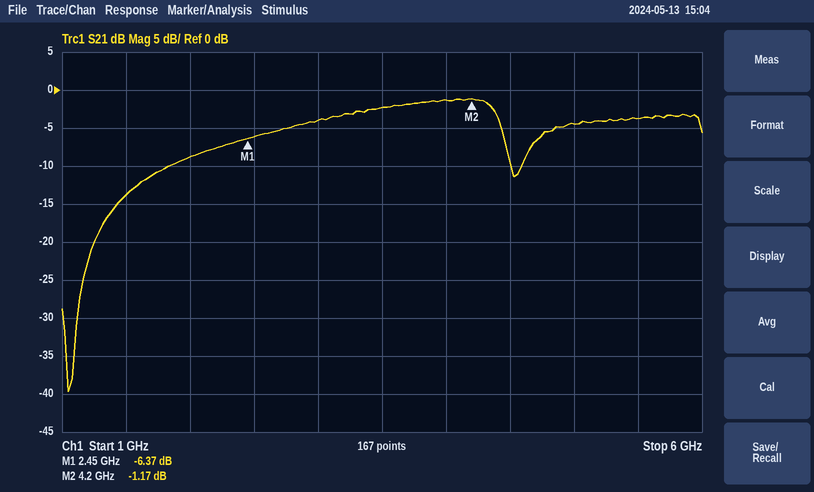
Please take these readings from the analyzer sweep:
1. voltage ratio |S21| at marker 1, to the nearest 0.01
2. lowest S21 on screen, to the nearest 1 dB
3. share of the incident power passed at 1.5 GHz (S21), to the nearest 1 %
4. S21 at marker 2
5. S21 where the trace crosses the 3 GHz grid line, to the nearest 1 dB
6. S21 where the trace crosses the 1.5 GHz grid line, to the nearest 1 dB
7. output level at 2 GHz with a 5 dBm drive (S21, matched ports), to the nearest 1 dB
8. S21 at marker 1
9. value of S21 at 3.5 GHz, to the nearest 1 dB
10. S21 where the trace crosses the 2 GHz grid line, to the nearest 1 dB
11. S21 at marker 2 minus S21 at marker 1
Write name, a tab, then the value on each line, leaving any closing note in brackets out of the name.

voltage ratio |S21| at marker 1, to the nearest 0.01	0.48
lowest S21 on screen, to the nearest 1 dB	-40 dB
share of the incident power passed at 1.5 GHz (S21), to the nearest 1 %	4 %
S21 at marker 2	-1.17 dB
S21 where the trace crosses the 3 GHz grid line, to the nearest 1 dB	-4 dB
S21 where the trace crosses the 1.5 GHz grid line, to the nearest 1 dB	-14 dB
output level at 2 GHz with a 5 dBm drive (S21, matched ports), to the nearest 1 dB	-4 dBm
S21 at marker 1	-6.37 dB
value of S21 at 3.5 GHz, to the nearest 1 dB	-2 dB
S21 where the trace crosses the 2 GHz grid line, to the nearest 1 dB	-9 dB
S21 at marker 2 minus S21 at marker 1	5.20 dB
